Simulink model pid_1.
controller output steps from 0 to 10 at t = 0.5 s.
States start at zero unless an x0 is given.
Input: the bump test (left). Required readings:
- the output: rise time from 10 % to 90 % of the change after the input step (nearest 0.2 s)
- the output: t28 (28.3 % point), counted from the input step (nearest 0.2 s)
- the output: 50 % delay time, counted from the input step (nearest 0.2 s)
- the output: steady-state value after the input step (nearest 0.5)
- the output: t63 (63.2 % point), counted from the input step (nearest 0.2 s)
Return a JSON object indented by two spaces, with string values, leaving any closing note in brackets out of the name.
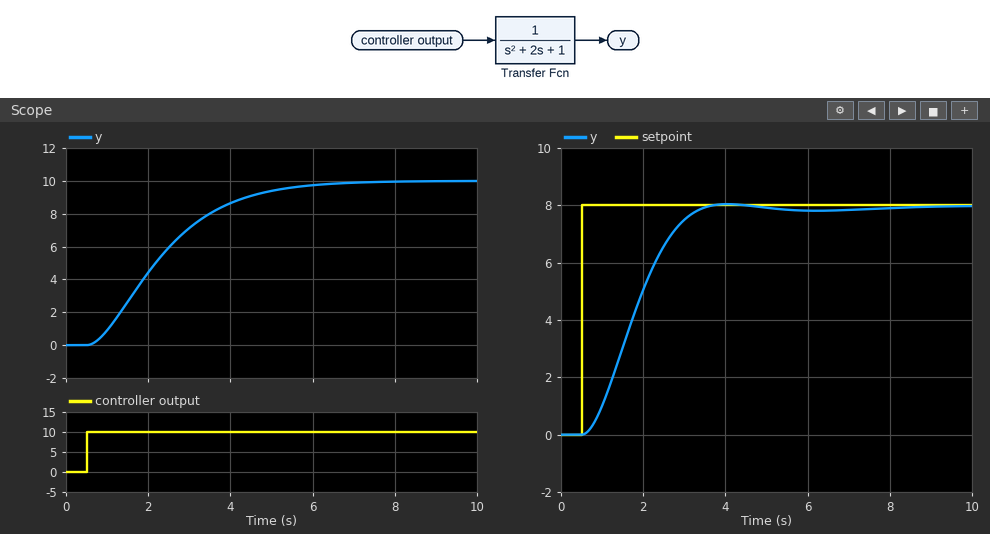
{
  "the output: rise time from 10 % to 90 % of the change after the input step": "3.4 s",
  "the output: t28 (28.3 % point), counted from the input step": "1.0 s",
  "the output: 50 % delay time, counted from the input step": "1.6 s",
  "the output: steady-state value after the input step": "10.0",
  "the output: t63 (63.2 % point), counted from the input step": "2.2 s"
}
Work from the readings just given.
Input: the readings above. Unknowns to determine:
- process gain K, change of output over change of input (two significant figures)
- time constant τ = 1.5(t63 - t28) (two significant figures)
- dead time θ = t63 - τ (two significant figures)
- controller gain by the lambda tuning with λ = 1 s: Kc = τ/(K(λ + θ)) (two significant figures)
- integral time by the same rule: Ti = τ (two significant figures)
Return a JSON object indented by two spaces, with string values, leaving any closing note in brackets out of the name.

{
  "process gain K, change of output over change of input": "1.0",
  "time constant τ = 1.5(t63 - t28)": "1.8 s",
  "dead time θ = t63 - τ": "0.40 s",
  "controller gain by the lambda tuning with λ = 1 s: Kc = τ/(K(λ + θ))": "1.3",
  "integral time by the same rule: Ti = τ": "1.8 s"
}
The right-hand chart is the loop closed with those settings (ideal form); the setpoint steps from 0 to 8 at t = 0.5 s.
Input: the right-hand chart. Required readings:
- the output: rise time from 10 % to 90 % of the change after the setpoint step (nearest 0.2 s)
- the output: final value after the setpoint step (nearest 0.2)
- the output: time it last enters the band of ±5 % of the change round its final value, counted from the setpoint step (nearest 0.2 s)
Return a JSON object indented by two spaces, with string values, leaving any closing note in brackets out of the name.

{
  "the output: rise time from 10 % to 90 % of the change after the setpoint step": "1.8 s",
  "the output: final value after the setpoint step": "8.0",
  "the output: time it last enters the band of ±5 % of the change round its final value, counted from the setpoint step": "2.6 s"
}
